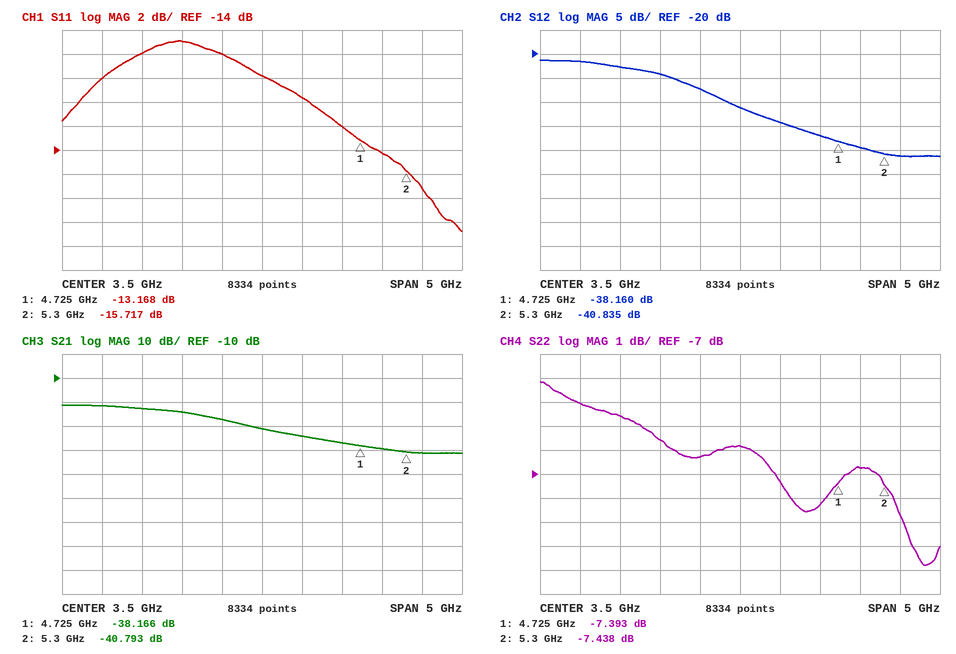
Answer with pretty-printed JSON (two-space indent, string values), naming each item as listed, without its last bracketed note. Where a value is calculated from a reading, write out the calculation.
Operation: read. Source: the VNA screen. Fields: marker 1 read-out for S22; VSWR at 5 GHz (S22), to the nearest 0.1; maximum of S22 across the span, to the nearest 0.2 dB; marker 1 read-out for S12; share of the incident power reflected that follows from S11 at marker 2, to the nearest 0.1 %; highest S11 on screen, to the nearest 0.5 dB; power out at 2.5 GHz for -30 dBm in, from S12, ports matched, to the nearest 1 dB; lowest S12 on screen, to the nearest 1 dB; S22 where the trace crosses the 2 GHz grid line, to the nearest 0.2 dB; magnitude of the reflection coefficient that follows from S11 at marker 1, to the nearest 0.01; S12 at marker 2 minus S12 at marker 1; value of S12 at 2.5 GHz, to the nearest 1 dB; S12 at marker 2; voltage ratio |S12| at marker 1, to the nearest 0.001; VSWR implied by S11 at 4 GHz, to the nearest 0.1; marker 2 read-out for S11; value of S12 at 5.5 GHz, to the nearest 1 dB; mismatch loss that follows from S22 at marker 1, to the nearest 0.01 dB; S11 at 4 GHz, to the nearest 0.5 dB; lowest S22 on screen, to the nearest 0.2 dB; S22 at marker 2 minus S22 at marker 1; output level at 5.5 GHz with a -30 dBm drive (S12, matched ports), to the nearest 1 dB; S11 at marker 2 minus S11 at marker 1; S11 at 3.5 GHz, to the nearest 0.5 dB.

{
  "marker 1 read-out for S22": "-7.393 dB",
  "VSWR at 5 GHz (S22), to the nearest 0.1": "|Γ| = 10^(-6.8/20) = 0.4571; VSWR = (1 + 0.4571)/(1 − 0.4571) ≈ 2.7",
  "maximum of S22 across the span, to the nearest 0.2 dB": "-3.2 dB",
  "marker 1 read-out for S12": "-38.160 dB",
  "share of the incident power reflected that follows from S11 at marker 2, to the nearest 0.1 %": "10^(-15.717/10) ≈ 2.7 %",
  "highest S11 on screen, to the nearest 0.5 dB": "-5.0 dB",
  "power out at 2.5 GHz for -30 dBm in, from S12, ports matched, to the nearest 1 dB": "-30 dBm + (-24 dB) = -54 dBm",
  "lowest S12 on screen, to the nearest 1 dB": "-41 dB",
  "S22 where the trace crosses the 2 GHz grid line, to the nearest 0.2 dB": "-4.6 dB",
  "magnitude of the reflection coefficient that follows from S11 at marker 1, to the nearest 0.01": "10^(-13.168/20) ≈ 0.22",
  "S12 at marker 2 minus S12 at marker 1": "-40.835 − (-38.16) = -2.675 dB",
  "value of S12 at 2.5 GHz, to the nearest 1 dB": "-24 dB",
  "S12 at marker 2": "-40.835 dB",
  "voltage ratio |S12| at marker 1, to the nearest 0.001": "10^(-38.16/20) ≈ 0.012",
  "VSWR implied by S11 at 4 GHz, to the nearest 0.1": "|Γ| = 10^(-9.5/20) = 0.3350; VSWR = (1 + 0.3350)/(1 − 0.3350) ≈ 2.0",
  "marker 2 read-out for S11": "-15.717 dB",
  "value of S12 at 5.5 GHz, to the nearest 1 dB": "-41 dB",
  "mismatch loss that follows from S22 at marker 1, to the nearest 0.01 dB": "−10 log10(1 − 10^(-7.393/10)) ≈ 0.87 dB",
  "S11 at 4 GHz, to the nearest 0.5 dB": "-9.5 dB",
  "lowest S22 on screen, to the nearest 0.2 dB": "-10.8 dB",
  "S22 at marker 2 minus S22 at marker 1": "-7.438 − (-7.393) = -0.045 dB",
  "output level at 5.5 GHz with a -30 dBm drive (S12, matched ports), to the nearest 1 dB": "-30 dBm + (-41 dB) = -71 dBm",
  "S11 at marker 2 minus S11 at marker 1": "-15.717 − (-13.168) = -2.549 dB",
  "S11 at 3.5 GHz, to the nearest 0.5 dB": "-8.0 dB"
}
